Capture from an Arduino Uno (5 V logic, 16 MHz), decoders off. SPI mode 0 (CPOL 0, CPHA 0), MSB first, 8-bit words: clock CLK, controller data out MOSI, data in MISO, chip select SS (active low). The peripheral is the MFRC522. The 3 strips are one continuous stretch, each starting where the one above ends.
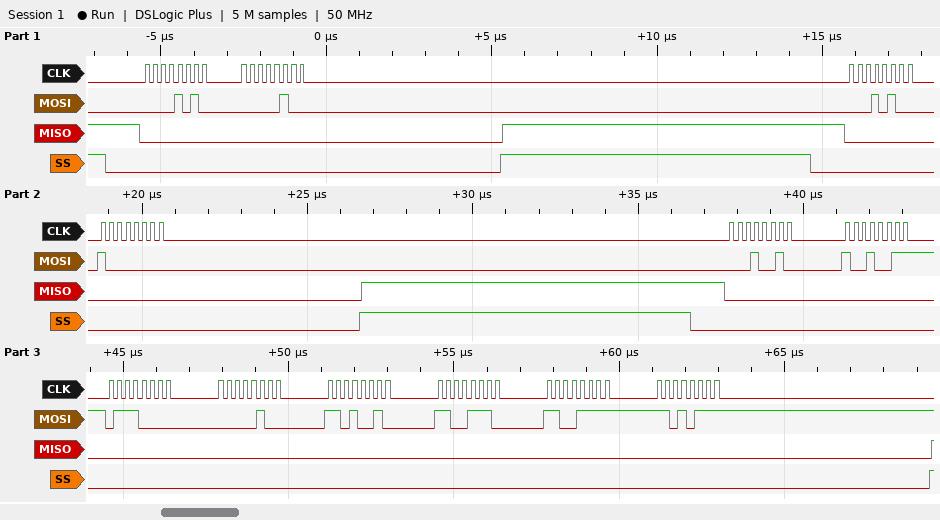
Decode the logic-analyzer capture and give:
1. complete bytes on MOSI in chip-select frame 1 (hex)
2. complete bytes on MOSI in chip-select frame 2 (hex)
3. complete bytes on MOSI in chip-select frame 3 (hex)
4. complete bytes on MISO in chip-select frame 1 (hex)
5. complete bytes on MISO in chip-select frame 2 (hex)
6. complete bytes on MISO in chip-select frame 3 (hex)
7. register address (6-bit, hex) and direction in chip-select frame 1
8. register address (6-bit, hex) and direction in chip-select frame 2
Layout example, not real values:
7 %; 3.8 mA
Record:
0A 04; 14 80; 12 93 70 04 D2 CE CF D7; 00 00; 00 00; 00 00 00 00 00 00 00 00; 0x05 write; 0x0A write
